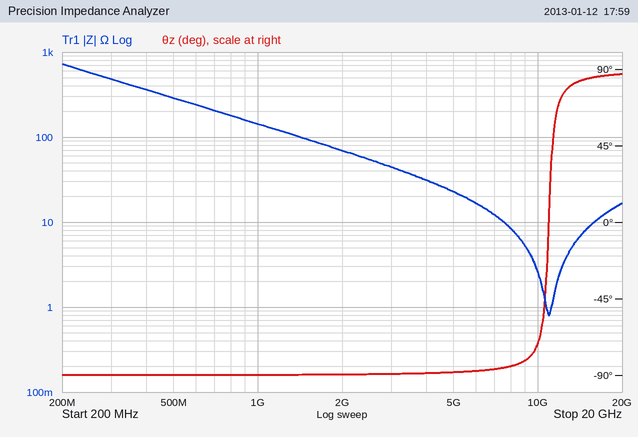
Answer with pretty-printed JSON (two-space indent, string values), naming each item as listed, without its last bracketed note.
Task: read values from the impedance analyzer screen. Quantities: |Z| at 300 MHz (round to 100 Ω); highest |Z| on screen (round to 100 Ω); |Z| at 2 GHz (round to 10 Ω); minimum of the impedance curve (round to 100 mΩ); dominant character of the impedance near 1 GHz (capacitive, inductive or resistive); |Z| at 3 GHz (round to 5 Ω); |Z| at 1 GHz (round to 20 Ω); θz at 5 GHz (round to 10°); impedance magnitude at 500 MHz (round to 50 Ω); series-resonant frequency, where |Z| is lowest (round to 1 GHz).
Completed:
{
  "|Z| at 300 MHz": "500 Ω",
  "highest |Z| on screen": "700 Ω",
  "|Z| at 2 GHz": "70 Ω",
  "minimum of the impedance curve": "800 mΩ",
  "dominant character of the impedance near 1 GHz": "capacitive",
  "|Z| at 3 GHz": "45 Ω",
  "|Z| at 1 GHz": "140 Ω",
  "θz at 5 GHz": "-90°",
  "impedance magnitude at 500 MHz": "300 Ω",
  "series-resonant frequency, where |Z| is lowest": "11 GHz"
}
